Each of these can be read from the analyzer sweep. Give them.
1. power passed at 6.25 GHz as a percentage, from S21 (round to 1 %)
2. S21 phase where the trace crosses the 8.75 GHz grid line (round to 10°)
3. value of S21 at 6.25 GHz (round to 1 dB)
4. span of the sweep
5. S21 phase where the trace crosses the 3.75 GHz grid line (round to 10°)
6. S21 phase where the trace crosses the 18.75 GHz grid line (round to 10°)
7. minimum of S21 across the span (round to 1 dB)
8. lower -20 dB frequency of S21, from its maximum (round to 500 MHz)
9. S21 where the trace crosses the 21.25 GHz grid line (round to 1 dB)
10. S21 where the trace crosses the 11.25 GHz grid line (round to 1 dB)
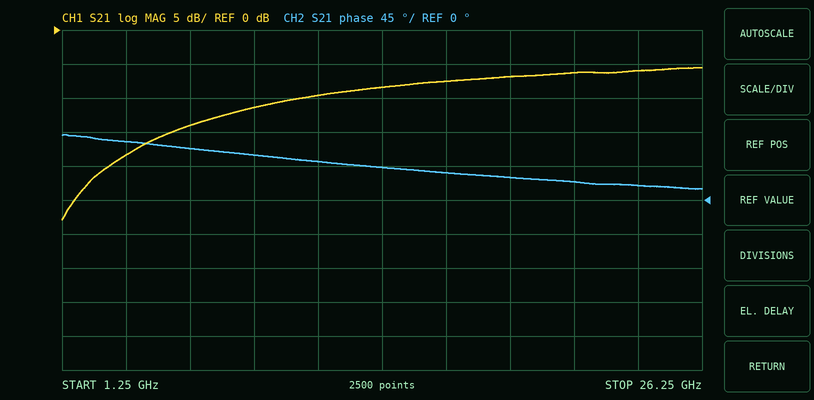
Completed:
4 %
60°
-14 dB
25 GHz
80°
30°
-28 dB
1.5 GHz
-6 dB
-10 dB
